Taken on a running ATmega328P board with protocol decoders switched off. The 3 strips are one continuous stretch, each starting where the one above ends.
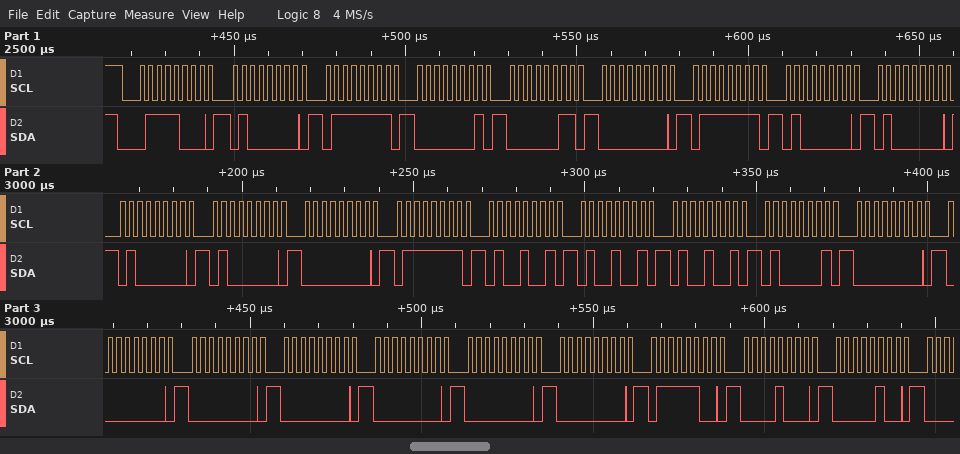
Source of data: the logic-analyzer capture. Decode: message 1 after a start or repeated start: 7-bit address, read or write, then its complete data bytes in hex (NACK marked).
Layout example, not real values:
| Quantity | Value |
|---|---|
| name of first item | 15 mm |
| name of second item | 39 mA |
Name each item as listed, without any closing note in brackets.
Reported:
| Quantity | Value |
|---|---|
| message 1 after a start or repeated start: 7-bit address, read or write, then its complete data bytes in hex | 0x3C write: 40 7F 01 03 00 7F 40 40 40 40 00 7F 49 49 49 41 00 00 00 00 00 00 00 7C 08 04 |
